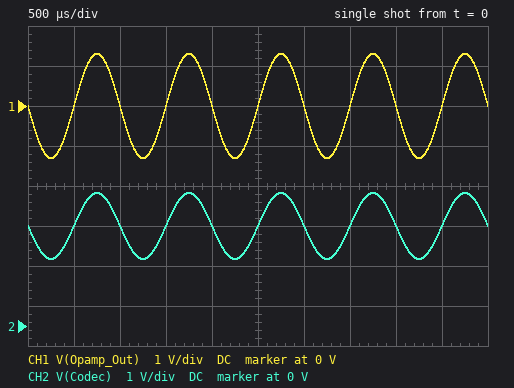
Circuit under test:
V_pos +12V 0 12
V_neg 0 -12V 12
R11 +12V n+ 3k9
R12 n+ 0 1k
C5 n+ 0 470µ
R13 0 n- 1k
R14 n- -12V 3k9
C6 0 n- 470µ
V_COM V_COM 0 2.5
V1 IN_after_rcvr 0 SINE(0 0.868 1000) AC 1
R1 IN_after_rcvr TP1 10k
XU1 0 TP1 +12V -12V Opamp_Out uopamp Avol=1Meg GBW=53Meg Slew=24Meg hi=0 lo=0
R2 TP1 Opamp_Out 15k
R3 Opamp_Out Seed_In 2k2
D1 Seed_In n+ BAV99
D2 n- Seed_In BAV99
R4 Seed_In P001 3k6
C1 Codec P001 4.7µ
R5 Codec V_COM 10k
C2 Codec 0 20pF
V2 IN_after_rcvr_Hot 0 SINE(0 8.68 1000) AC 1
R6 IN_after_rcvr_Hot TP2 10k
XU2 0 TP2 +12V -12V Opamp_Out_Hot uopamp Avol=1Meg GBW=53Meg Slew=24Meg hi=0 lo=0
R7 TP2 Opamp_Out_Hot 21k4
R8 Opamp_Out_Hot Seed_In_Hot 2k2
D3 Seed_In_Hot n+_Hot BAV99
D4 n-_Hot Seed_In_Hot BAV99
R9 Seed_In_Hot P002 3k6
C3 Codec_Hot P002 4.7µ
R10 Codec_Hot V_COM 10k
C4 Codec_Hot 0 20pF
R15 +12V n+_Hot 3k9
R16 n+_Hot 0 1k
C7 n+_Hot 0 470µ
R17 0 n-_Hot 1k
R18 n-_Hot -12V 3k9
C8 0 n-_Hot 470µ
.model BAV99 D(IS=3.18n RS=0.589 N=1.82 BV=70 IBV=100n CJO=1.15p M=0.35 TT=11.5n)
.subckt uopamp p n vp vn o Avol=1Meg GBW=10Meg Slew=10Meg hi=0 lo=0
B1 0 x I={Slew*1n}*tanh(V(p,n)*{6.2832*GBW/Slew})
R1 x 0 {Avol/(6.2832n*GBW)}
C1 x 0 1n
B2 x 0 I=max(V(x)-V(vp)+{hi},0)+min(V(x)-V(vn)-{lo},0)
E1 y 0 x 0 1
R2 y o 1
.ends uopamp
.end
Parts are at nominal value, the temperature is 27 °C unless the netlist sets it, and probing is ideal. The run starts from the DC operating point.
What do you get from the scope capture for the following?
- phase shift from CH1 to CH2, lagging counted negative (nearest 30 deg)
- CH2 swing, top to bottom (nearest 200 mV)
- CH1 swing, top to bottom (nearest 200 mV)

0 deg
1.6 V
2.6 V
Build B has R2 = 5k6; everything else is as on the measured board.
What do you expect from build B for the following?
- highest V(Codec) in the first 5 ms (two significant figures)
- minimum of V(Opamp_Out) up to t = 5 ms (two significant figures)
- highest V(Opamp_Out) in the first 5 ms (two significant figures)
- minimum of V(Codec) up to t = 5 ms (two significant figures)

2.8 V
-490 mV
490 mV
2.2 V
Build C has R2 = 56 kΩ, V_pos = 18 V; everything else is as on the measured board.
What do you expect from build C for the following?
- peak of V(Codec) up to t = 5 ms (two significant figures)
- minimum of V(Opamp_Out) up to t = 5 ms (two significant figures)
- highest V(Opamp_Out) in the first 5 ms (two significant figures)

5.5 V
-4.9 V
4.9 V
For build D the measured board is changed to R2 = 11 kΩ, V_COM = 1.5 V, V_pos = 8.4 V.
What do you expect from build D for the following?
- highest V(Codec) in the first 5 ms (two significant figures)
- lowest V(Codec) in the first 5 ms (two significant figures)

2.1 V
900 mV
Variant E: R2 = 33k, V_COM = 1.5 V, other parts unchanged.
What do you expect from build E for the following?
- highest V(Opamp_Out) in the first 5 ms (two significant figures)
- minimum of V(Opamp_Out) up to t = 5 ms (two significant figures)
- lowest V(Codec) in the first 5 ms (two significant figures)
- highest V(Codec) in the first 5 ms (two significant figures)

2.9 V
-2.9 V
-310 mV
3.3 V
